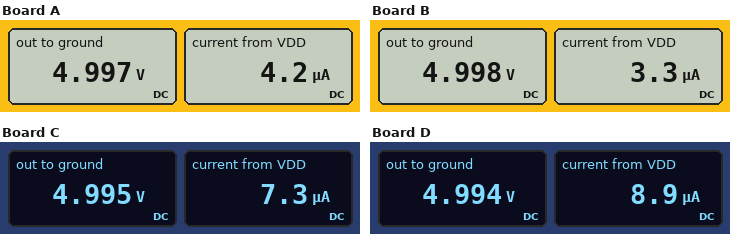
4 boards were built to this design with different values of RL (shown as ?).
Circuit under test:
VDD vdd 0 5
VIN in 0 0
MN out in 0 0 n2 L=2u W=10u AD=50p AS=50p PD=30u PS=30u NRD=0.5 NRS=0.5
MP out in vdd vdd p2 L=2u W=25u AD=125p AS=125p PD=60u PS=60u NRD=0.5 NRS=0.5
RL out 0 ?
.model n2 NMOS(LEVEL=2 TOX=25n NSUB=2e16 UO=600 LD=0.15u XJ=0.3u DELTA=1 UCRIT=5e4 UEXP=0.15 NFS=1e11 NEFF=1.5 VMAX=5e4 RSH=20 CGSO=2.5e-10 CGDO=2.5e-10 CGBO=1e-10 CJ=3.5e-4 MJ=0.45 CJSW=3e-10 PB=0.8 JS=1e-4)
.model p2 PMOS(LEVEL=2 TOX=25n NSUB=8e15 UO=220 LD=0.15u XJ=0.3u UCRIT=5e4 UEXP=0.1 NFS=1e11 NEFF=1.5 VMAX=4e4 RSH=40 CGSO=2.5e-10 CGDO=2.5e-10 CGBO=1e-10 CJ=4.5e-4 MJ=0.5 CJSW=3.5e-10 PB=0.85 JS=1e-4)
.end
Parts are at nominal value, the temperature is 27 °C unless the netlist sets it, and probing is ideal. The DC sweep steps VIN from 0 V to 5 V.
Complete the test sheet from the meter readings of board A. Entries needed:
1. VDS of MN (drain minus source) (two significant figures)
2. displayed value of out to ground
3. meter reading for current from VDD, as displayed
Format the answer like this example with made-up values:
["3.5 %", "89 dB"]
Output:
["5.0 V", "4.997 V", "4.2 µA"]
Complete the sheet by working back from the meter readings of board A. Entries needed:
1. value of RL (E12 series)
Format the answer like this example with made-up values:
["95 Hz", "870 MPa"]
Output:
["1.2 MΩ"]
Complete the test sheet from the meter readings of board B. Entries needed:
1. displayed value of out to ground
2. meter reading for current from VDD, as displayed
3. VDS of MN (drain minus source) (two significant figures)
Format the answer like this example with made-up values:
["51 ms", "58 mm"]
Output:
["4.998 V", "3.3 µA", "5.0 V"]
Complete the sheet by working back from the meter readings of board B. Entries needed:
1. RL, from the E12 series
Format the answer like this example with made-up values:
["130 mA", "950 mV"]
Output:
["1.5 MΩ"]
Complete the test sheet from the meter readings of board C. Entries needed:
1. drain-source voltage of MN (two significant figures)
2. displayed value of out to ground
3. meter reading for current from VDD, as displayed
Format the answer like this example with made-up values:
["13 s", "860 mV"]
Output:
["5.0 V", "4.995 V", "7.3 µA"]
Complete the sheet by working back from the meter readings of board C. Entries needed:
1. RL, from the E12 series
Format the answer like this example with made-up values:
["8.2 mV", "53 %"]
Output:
["680 kΩ"]
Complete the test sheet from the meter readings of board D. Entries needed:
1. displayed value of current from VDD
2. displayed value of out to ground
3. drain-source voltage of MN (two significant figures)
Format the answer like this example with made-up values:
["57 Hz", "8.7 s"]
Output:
["8.9 µA", "4.994 V", "5.0 V"]
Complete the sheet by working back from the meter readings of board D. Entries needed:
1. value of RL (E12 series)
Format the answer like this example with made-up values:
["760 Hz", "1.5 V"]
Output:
["560 kΩ"]
